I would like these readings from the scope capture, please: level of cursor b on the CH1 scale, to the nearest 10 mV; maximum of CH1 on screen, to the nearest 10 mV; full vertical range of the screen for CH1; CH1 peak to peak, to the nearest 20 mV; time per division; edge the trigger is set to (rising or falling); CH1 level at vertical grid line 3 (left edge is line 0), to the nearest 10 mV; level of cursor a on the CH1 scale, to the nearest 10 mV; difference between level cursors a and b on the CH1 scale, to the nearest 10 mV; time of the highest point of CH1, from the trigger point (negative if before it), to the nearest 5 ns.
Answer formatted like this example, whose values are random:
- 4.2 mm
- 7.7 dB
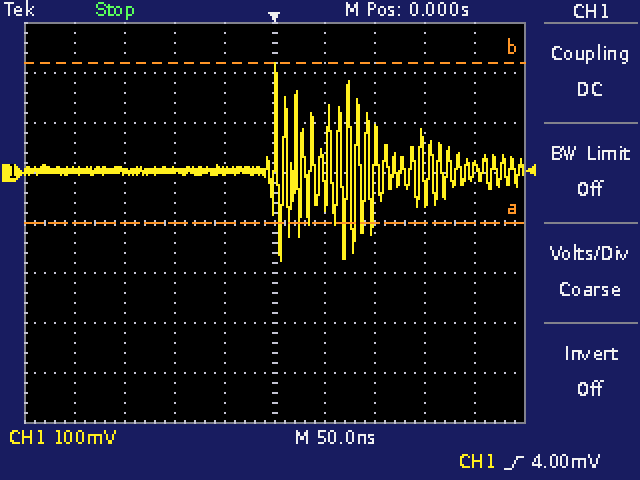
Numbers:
- 220 mV
- 220 mV
- 800 mV
- 400 mV
- 50 ns
- rising
- 10 mV
- -100 mV
- 320 mV
- 0 ns
